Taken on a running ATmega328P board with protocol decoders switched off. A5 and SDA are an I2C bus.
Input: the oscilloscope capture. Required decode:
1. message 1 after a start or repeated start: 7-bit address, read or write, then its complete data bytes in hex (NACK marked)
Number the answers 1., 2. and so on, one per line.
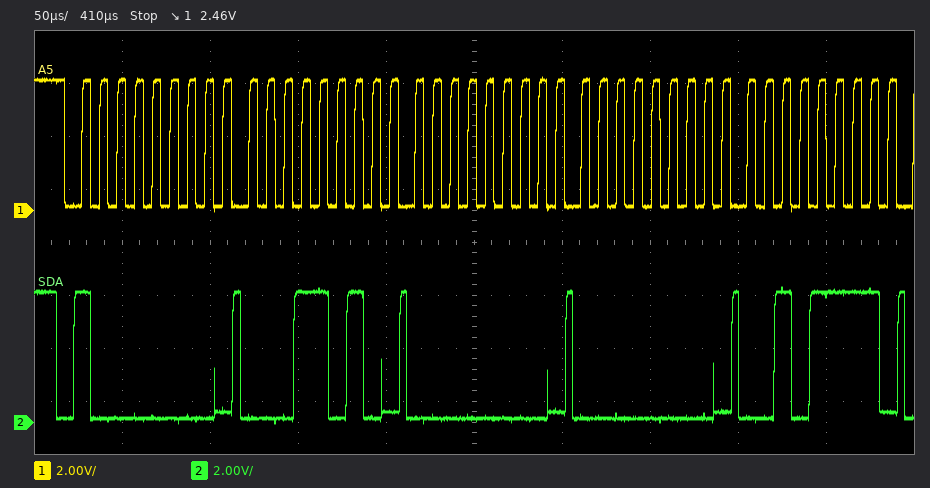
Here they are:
1. 0x40 write: 1A 00 00 2F
